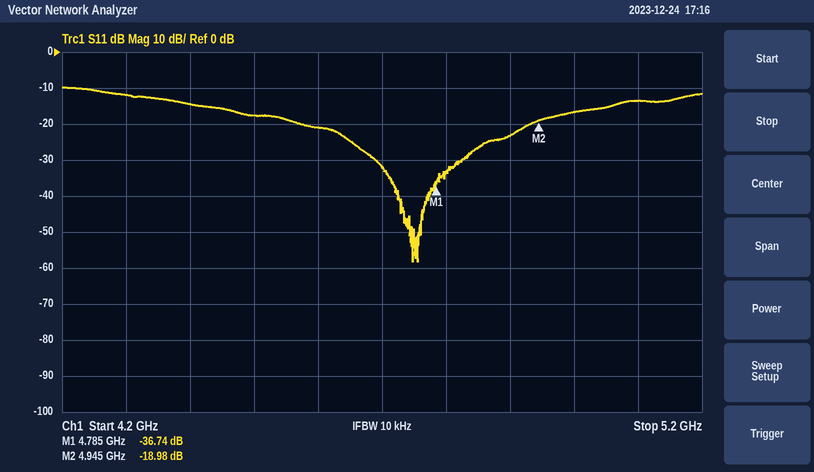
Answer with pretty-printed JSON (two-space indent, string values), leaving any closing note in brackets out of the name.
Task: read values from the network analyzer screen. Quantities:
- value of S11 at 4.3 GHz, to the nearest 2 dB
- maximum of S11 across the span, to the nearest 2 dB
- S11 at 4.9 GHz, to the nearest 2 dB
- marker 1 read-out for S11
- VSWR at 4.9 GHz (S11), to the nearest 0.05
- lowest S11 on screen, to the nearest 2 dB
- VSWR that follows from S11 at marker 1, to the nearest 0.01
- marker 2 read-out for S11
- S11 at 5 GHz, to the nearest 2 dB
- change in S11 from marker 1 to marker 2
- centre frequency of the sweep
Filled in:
{
  "value of S11 at 4.3 GHz, to the nearest 2 dB": "-12 dB",
  "maximum of S11 across the span, to the nearest 2 dB": "-10 dB",
  "S11 at 4.9 GHz, to the nearest 2 dB": "-24 dB",
  "marker 1 read-out for S11": "-36.74 dB",
  "VSWR at 4.9 GHz (S11), to the nearest 0.05": "1.15",
  "lowest S11 on screen, to the nearest 2 dB": "-58 dB",
  "VSWR that follows from S11 at marker 1, to the nearest 0.01": "1.03",
  "marker 2 read-out for S11": "-18.98 dB",
  "S11 at 5 GHz, to the nearest 2 dB": "-16 dB",
  "change in S11 from marker 1 to marker 2": "17.76 dB",
  "centre frequency of the sweep": "4.7 GHz"
}
